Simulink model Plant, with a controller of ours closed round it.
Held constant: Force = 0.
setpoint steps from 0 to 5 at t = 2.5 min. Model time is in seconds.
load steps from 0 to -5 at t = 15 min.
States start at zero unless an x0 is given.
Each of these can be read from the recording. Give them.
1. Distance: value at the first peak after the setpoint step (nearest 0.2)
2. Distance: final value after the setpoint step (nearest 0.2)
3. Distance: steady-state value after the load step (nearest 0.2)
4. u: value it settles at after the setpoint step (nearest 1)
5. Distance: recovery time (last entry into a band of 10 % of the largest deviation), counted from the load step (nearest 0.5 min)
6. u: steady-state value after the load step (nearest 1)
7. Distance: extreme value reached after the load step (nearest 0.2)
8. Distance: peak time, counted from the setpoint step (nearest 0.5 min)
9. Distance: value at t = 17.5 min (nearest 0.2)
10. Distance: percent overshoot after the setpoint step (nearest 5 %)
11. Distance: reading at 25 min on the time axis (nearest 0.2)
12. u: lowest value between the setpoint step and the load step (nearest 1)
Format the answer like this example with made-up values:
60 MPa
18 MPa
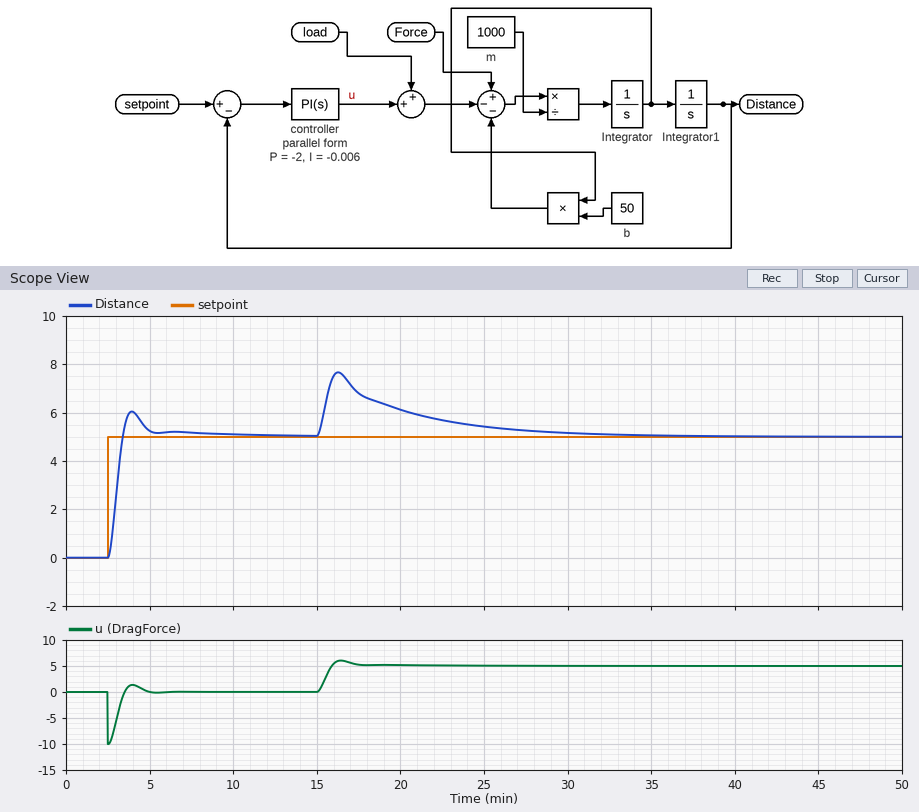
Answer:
6.0
5.0
5.0
0
12.5 min
5
7.6
1.5 min
6.8
20 %
5.4
-10
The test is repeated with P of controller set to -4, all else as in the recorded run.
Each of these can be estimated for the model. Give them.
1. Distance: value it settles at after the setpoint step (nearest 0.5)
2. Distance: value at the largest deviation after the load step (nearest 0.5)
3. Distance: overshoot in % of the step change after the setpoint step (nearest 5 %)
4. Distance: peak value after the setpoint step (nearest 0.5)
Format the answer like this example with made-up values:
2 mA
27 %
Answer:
5.0
6.5
30 %
6.5
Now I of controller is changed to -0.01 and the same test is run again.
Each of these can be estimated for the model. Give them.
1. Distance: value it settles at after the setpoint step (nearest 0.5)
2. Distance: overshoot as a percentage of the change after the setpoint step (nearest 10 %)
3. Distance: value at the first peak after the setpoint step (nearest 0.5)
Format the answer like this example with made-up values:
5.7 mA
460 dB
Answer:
5.0
30 %
6.5
